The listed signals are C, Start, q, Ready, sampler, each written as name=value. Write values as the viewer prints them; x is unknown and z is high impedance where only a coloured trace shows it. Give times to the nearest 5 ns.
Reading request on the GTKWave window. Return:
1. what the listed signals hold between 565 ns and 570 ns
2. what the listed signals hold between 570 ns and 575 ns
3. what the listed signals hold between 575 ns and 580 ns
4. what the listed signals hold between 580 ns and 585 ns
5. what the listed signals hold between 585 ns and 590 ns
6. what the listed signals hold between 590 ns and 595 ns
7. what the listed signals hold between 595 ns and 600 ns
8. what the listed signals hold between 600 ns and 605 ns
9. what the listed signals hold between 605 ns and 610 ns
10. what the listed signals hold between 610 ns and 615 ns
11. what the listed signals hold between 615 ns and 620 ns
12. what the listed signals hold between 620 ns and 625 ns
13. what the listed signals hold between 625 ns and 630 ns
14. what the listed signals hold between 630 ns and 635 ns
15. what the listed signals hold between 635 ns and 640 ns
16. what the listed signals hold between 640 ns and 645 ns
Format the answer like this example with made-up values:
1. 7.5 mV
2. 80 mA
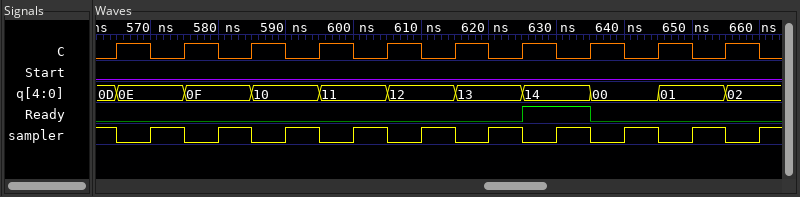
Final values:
1. C=1, Start=0, q=0E, Ready=0, sampler=0
2. C=0, Start=0, q=0E, Ready=0, sampler=1
3. C=1, Start=0, q=0F, Ready=0, sampler=0
4. C=0, Start=0, q=0F, Ready=0, sampler=1
5. C=1, Start=0, q=10, Ready=0, sampler=0
6. C=0, Start=0, q=10, Ready=0, sampler=1
7. C=1, Start=0, q=11, Ready=0, sampler=0
8. C=0, Start=0, q=11, Ready=0, sampler=1
9. C=1, Start=0, q=12, Ready=0, sampler=0
10. C=0, Start=0, q=12, Ready=0, sampler=1
11. C=1, Start=0, q=13, Ready=0, sampler=0
12. C=0, Start=0, q=13, Ready=0, sampler=1
13. C=1, Start=0, q=14, Ready=1, sampler=0
14. C=0, Start=0, q=14, Ready=1, sampler=1
15. C=1, Start=0, q=00, Ready=0, sampler=0
16. C=0, Start=0, q=00, Ready=0, sampler=1
